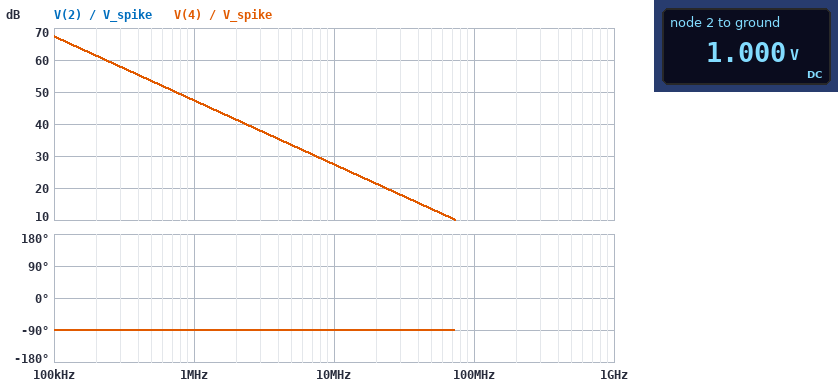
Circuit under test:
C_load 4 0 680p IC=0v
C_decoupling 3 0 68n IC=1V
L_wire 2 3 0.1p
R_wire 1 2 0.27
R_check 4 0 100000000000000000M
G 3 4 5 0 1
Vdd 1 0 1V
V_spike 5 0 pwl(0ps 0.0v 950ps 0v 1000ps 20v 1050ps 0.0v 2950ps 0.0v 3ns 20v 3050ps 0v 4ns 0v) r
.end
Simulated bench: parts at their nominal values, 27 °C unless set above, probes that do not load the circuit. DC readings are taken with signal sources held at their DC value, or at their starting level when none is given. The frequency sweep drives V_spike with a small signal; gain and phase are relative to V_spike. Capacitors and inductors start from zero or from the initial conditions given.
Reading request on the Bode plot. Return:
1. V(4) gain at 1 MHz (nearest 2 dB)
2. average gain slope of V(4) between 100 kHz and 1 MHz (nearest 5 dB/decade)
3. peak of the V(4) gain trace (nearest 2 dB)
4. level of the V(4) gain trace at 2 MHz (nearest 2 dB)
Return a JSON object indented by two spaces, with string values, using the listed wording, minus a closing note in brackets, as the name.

{
  "V(4) gain at 1 MHz": "48 dB",
  "average gain slope of V(4) between 100 kHz and 1 MHz": "-20 dB/decade",
  "peak of the V(4) gain trace": "68 dB",
  "level of the V(4) gain trace at 2 MHz": "42 dB"
}
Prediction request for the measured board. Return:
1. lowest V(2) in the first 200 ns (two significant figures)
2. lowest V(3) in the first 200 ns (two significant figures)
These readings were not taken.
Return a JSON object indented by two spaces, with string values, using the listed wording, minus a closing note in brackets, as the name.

{
  "lowest V(2) in the first 200 ns": "860 mV",
  "lowest V(3) in the first 200 ns": "860 mV"
}
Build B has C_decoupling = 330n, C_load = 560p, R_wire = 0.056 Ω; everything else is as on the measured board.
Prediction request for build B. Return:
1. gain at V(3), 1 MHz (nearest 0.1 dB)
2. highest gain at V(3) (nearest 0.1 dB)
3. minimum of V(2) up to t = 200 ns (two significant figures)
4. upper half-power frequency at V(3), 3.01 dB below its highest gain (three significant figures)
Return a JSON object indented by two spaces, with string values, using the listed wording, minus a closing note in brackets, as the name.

{
  "gain at V(3), 1 MHz": "-25.1 dB",
  "highest gain at V(3)": "-25.0 dB",
  "minimum of V(2) up to t = 200 ns": "970 mV",
  "upper half-power frequency at V(3), 3.01 dB below its highest gain": "8.61 MHz"
}
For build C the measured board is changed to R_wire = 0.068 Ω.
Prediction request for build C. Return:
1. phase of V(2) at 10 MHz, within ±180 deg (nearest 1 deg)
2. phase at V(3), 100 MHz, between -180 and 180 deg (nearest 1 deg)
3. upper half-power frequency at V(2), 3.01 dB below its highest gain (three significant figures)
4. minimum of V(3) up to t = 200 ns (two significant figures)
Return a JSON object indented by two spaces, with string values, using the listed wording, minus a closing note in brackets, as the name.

{
  "phase of V(2) at 10 MHz, within ±180 deg": "164 deg",
  "phase at V(3), 100 MHz, between -180 and 180 deg": "109 deg",
  "upper half-power frequency at V(2), 3.01 dB below its highest gain": "34.4 MHz",
  "minimum of V(3) up to t = 200 ns": "960 mV"
}
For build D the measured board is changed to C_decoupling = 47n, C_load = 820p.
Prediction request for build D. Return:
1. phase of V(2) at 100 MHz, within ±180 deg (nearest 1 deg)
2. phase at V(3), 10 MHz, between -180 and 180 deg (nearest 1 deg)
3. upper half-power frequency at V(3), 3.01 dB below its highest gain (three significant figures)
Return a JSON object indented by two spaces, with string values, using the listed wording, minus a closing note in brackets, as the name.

{
  "phase of V(2) at 100 MHz, within ±180 deg": "97 deg",
  "phase at V(3), 10 MHz, between -180 and 180 deg": "141 deg",
  "upper half-power frequency at V(3), 3.01 dB below its highest gain": "12.5 MHz"
}
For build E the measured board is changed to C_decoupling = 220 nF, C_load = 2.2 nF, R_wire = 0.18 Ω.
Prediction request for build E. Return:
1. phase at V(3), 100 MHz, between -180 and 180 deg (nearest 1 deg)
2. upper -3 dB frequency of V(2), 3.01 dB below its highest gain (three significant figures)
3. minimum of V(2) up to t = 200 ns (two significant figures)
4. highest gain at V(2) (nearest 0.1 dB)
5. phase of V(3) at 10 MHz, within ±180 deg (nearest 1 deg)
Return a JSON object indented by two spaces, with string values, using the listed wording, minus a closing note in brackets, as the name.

{
  "phase at V(3), 100 MHz, between -180 and 180 deg": "92 deg",
  "upper -3 dB frequency of V(2), 3.01 dB below its highest gain": "4.02 MHz",
  "minimum of V(2) up to t = 200 ns": "910 mV",
  "highest gain at V(2)": "-14.9 dB",
  "phase of V(3) at 10 MHz, within ±180 deg": "112 deg"
}
